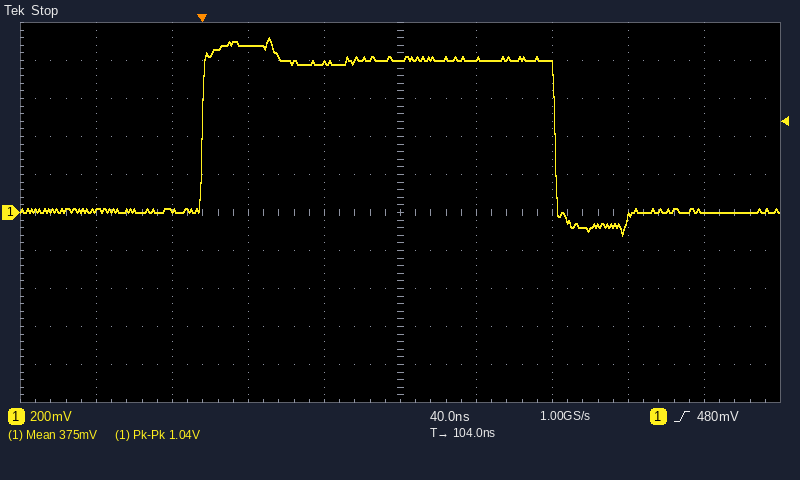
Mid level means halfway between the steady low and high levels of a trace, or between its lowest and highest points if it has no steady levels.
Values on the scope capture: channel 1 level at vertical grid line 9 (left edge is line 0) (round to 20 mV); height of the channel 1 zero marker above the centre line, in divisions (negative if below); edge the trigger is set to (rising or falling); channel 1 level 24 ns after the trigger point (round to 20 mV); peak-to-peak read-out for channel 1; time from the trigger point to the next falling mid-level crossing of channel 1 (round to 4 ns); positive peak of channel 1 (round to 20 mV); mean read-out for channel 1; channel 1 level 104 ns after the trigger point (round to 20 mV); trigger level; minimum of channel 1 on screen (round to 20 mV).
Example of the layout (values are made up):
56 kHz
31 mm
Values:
0 mV
0.0 div
rising
880 mV
1.04 V
184 ns
920 mV
375 mV
800 mV
480 mV
-120 mV
